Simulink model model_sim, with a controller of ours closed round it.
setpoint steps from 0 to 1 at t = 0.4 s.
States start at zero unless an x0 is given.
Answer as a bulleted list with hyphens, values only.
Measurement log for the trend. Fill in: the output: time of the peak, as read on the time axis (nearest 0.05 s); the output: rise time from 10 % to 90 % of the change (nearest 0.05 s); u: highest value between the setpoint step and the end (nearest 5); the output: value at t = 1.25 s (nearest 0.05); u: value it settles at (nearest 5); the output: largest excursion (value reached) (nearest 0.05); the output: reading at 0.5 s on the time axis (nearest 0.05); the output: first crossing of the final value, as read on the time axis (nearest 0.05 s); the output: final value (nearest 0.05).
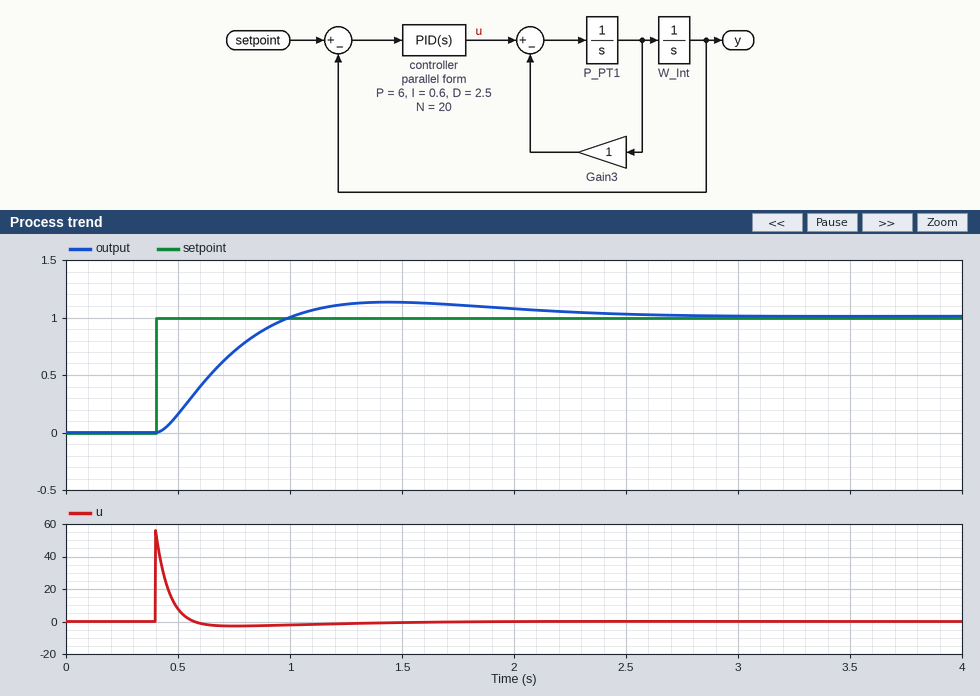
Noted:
- 1.45 s
- 0.40 s
- 55
- 1.10
- 0
- 1.15
- 0.15
- 1.00 s
- 1.00
